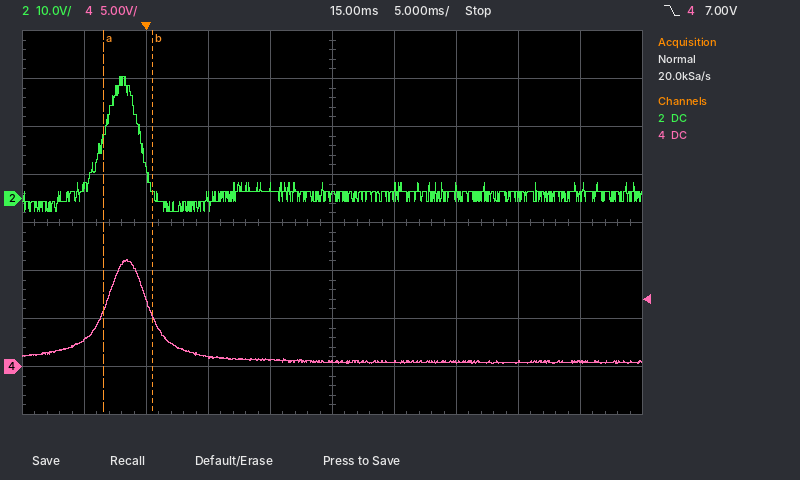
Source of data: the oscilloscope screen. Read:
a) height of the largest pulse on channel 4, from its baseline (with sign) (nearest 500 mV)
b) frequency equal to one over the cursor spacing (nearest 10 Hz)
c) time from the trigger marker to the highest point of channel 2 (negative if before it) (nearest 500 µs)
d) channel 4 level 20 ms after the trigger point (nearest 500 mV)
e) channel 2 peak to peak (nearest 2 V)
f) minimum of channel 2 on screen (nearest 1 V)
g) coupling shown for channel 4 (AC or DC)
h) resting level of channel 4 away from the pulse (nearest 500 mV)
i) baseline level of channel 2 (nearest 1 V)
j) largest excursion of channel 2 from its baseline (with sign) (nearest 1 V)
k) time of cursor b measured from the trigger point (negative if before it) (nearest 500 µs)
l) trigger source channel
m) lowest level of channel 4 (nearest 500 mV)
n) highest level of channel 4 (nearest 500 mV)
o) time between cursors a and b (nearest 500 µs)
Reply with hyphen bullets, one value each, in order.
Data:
- +10.5 V
- 250 Hz
- -2.0 ms
- 500 mV
- 28 V
- -3 V
- DC
- 500 mV
- 1 V
- +25 V
- +500 µs
- channel 4
- 500 mV
- 11.0 V
- 4.0 ms
